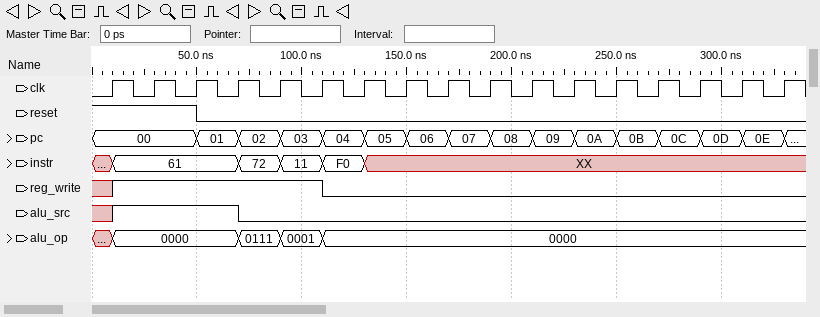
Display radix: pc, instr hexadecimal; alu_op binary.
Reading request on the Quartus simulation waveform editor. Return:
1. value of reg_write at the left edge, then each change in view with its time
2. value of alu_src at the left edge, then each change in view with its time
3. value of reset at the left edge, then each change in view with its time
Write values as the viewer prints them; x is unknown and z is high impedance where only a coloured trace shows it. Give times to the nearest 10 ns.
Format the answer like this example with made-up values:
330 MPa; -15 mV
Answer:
x, 1 at 10 ns, 0 at 110 ns; x, 1 at 10 ns, 0 at 70 ns; 1, 0 at 50 ns
